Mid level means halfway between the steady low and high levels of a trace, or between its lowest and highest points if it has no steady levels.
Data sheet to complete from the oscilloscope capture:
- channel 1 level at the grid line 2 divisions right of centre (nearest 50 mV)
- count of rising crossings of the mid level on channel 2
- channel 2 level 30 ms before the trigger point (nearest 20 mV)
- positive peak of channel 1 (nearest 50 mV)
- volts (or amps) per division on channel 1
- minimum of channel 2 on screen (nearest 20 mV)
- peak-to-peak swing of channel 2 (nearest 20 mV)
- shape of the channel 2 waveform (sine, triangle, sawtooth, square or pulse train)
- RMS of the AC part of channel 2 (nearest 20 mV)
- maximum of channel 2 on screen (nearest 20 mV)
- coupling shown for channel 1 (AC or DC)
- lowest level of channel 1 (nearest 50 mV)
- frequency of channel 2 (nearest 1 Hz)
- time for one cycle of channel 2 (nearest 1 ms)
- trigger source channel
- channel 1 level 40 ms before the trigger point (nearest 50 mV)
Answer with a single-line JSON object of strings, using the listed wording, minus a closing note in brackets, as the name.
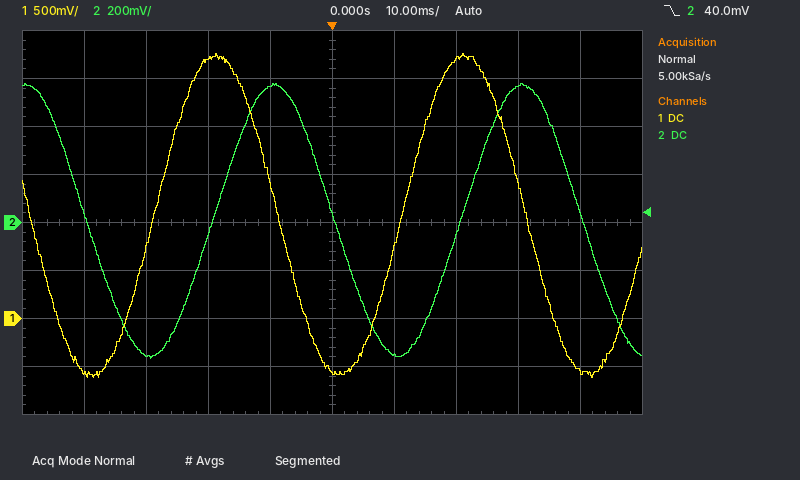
{"channel 1 level at the grid line 2 divisions right of centre": "2.70 V", "count of rising crossings of the mid level on channel 2": "2", "channel 2 level 30 ms before the trigger point": "-560 mV", "positive peak of channel 1": "2.75 V", "volts (or amps) per division on channel 1": "500 mV", "minimum of channel 2 on screen": "-560 mV", "peak-to-peak swing of channel 2": "1.14 V", "shape of the channel 2 waveform": "sine", "RMS of the AC part of channel 2": "400 mV", "maximum of channel 2 on screen": "580 mV", "coupling shown for channel 1": "DC", "lowest level of channel 1": "-600 mV", "frequency of channel 2": "25 Hz", "time for one cycle of channel 2": "40 ms", "trigger source channel": "channel 2", "channel 1 level 40 ms before the trigger point": "-550 mV"}
